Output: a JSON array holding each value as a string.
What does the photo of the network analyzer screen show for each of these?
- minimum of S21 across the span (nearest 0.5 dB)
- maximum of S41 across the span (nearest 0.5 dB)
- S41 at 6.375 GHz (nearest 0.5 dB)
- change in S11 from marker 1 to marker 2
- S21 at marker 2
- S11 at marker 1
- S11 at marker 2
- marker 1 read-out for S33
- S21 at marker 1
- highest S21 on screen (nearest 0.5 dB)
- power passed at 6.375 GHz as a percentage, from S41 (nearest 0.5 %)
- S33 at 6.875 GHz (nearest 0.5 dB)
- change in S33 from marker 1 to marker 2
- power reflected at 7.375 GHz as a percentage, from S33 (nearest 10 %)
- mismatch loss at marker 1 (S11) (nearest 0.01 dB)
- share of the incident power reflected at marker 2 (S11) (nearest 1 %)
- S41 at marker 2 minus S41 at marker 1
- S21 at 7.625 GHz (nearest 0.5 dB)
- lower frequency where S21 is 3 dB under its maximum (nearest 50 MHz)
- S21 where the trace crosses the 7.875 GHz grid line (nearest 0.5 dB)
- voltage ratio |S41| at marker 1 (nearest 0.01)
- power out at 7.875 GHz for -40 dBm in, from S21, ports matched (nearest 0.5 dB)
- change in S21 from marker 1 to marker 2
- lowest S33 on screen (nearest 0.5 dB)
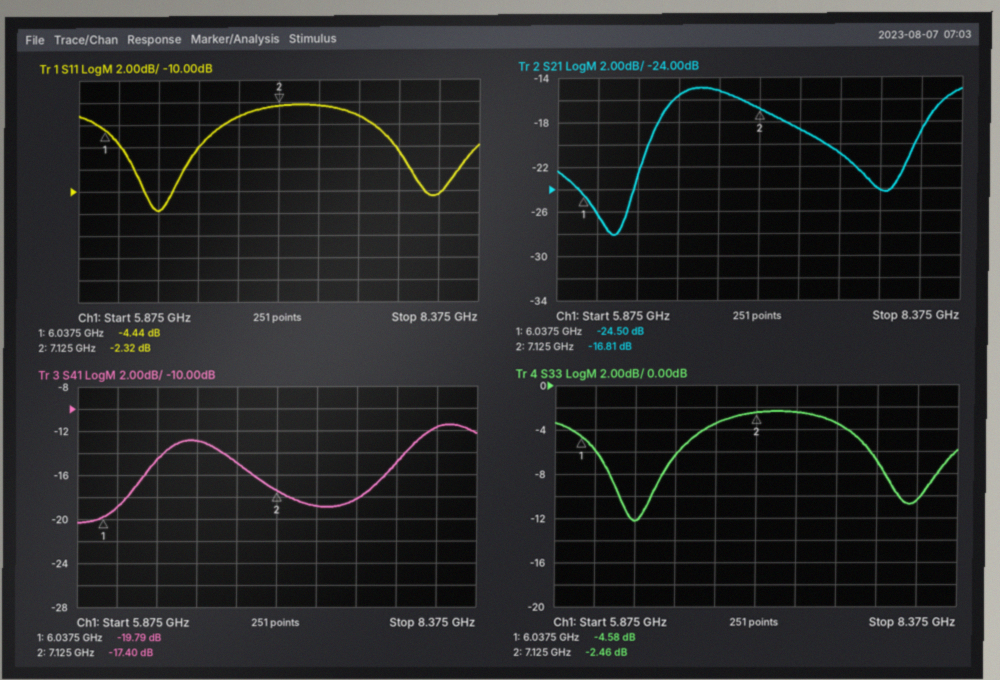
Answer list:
["-28.0 dB", "-11.5 dB", "-14.5 dB", "2.12 dB", "-16.81 dB", "-4.44 dB", "-2.32 dB", "-4.58 dB", "-24.50 dB", "-15.0 dB", "3.5 %", "-3.5 dB", "2.12 dB", "60 %", "1.94 dB", "59 %", "2.39 dB", "-21.0 dB", "6.50 GHz", "-24.0 dB", "0.10", "-64.0 dBm", "7.69 dB", "-12.0 dB"]
